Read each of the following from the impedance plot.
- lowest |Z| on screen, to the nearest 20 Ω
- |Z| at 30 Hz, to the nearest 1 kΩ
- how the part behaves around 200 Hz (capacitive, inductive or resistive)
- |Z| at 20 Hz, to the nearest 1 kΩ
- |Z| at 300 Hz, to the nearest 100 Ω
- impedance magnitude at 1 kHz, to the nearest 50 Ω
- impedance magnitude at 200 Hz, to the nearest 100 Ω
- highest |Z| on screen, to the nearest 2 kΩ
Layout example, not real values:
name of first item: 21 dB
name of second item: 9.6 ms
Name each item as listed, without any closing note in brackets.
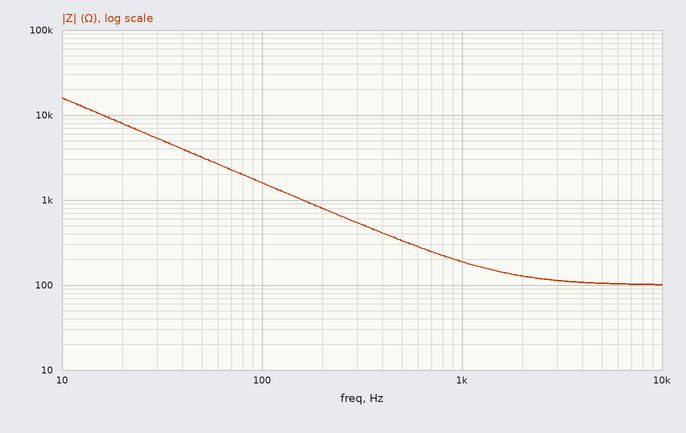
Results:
lowest |Z| on screen, to the nearest 20 Ω: 100 Ω
|Z| at 30 Hz, to the nearest 1 kΩ: 5 kΩ
how the part behaves around 200 Hz: capacitive
|Z| at 20 Hz, to the nearest 1 kΩ: 8 kΩ
|Z| at 300 Hz, to the nearest 100 Ω: 500 Ω
impedance magnitude at 1 kHz, to the nearest 50 Ω: 200 Ω
impedance magnitude at 200 Hz, to the nearest 100 Ω: 800 Ω
highest |Z| on screen, to the nearest 2 kΩ: 16 kΩ
